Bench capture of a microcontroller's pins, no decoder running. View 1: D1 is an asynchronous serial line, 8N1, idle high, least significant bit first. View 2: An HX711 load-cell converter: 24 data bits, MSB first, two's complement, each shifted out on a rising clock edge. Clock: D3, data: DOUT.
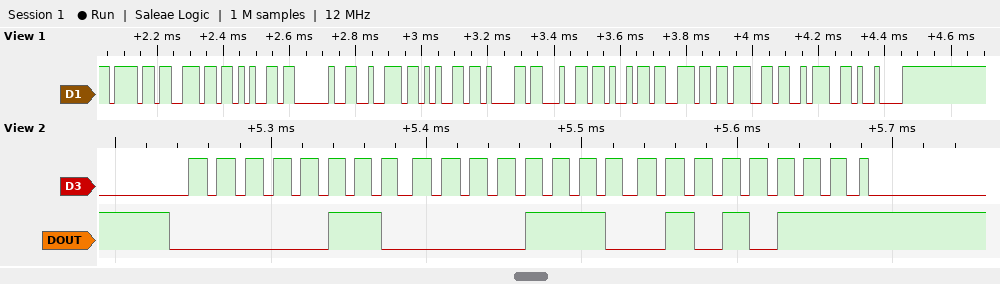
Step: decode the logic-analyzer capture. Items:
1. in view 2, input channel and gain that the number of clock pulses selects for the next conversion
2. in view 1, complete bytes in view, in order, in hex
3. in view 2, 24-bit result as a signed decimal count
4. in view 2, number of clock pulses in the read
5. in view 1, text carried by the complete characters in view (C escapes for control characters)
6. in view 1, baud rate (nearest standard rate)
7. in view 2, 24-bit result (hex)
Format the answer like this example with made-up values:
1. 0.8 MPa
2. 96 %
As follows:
1. channel A, gain 128
2. 6F 6E 65 20 72 65 61 64 69 6E 67 3A 09
3. 396887
4. 25
5. "one reading:\t"
6. 57600 baud
7. 0x060E57
